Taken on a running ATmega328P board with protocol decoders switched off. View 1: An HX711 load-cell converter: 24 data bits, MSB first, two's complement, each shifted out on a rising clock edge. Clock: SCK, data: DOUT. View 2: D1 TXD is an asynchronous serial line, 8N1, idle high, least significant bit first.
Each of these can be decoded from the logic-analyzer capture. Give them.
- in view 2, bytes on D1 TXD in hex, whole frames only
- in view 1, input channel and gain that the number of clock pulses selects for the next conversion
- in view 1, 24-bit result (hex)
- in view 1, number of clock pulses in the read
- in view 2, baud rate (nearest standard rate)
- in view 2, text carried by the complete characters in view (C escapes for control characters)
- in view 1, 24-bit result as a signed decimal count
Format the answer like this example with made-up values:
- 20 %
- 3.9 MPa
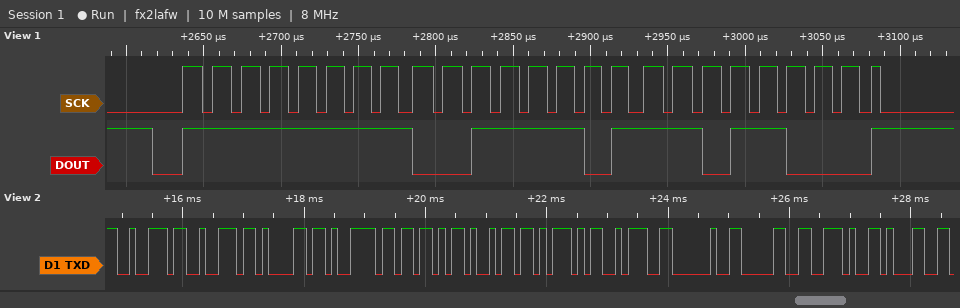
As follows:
- 72 72 61 79 5B 69 5D 3A 20 30 2E 31
- channel A, gain 128
- 0xFF3DD8
- 25
- 9600 baud
- "rray[i]: 0.1"
- -49704
